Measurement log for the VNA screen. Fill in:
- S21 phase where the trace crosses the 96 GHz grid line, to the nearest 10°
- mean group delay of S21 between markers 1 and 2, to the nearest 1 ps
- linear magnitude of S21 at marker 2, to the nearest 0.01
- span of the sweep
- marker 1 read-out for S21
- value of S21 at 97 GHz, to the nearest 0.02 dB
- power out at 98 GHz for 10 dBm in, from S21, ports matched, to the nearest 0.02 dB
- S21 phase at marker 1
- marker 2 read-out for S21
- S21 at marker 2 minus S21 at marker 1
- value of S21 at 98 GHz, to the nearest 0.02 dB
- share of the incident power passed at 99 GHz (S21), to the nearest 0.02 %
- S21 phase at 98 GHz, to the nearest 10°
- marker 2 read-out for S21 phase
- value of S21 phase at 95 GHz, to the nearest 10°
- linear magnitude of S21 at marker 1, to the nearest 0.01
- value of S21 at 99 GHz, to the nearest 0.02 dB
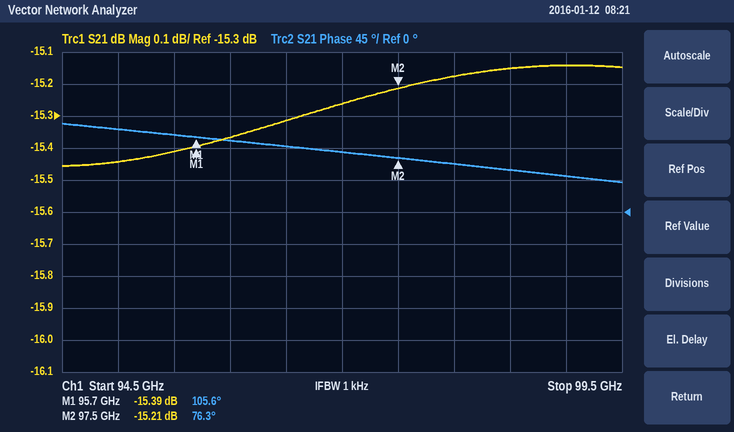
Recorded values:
100°
45 ps
0.17
5 GHz
-15.39 dB
-15.26 dB
-5.18 dBm
105.6°
-15.21 dB
0.18 dB
-15.18 dB
3.06 %
70°
76.3°
120°
0.17
-15.14 dB
